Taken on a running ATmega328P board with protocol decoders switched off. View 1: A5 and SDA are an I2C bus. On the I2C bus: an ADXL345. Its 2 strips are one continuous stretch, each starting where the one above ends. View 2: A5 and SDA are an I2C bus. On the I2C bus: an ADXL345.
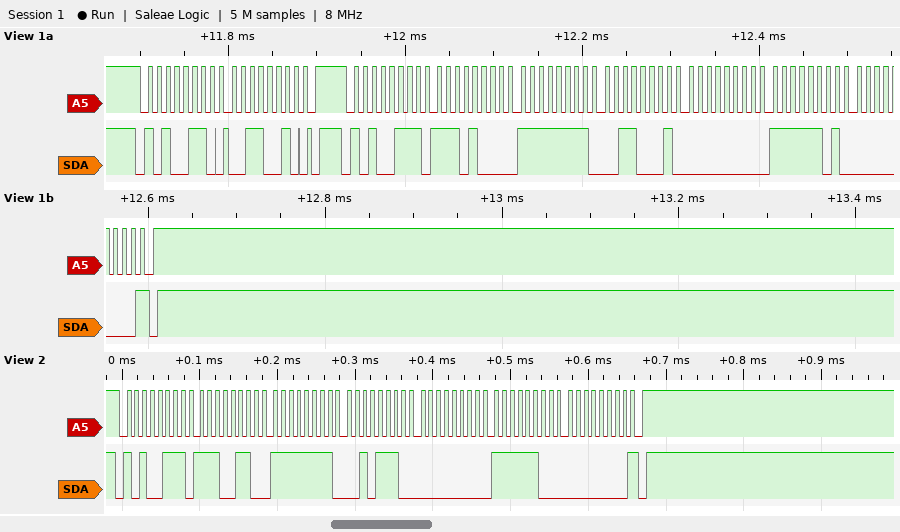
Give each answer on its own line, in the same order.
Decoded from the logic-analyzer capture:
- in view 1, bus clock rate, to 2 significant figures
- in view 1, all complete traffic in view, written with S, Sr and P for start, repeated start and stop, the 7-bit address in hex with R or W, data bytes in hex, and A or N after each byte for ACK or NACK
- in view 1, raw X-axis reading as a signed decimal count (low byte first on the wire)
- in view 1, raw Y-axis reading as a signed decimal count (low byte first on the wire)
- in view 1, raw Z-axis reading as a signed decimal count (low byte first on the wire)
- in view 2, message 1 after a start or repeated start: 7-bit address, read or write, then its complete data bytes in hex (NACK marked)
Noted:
100 kHz
S 53W A 32 A P S 53R A E8 A FF A 31 A 00 A FD A 00 N P
-24
49
253
0x53 read: E6 FF 2E 00 FC 00 NACK
